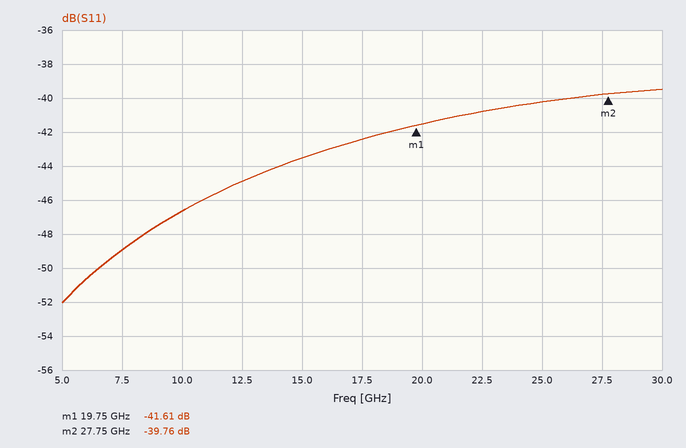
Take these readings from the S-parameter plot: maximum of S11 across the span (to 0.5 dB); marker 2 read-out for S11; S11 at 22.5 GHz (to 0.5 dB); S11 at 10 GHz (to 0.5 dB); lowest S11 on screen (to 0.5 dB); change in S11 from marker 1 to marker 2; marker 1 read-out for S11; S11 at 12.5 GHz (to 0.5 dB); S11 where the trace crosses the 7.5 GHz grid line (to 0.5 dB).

-39.5 dB
-39.76 dB
-41.0 dB
-46.5 dB
-52.0 dB
1.85 dB
-41.61 dB
-45.0 dB
-49.0 dB
